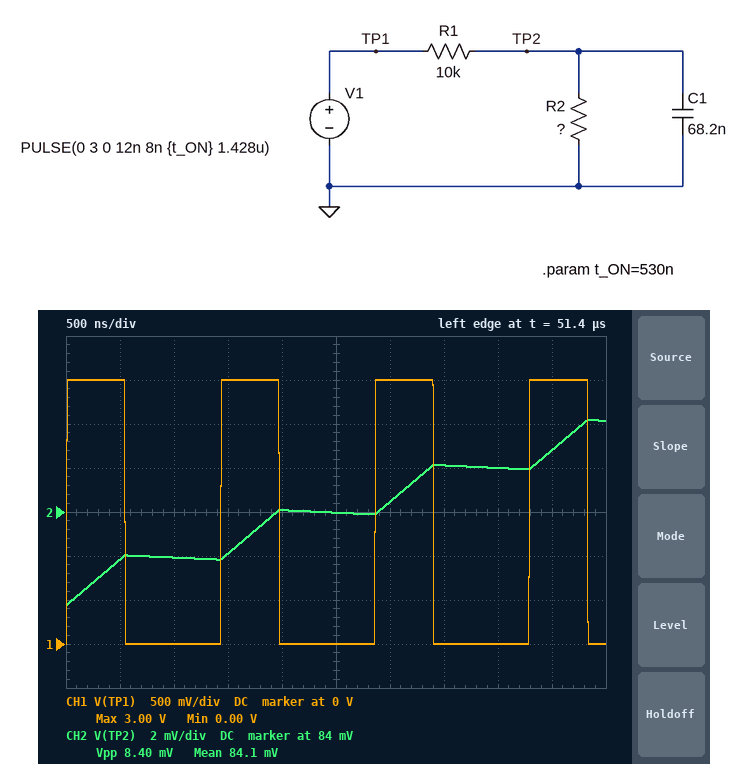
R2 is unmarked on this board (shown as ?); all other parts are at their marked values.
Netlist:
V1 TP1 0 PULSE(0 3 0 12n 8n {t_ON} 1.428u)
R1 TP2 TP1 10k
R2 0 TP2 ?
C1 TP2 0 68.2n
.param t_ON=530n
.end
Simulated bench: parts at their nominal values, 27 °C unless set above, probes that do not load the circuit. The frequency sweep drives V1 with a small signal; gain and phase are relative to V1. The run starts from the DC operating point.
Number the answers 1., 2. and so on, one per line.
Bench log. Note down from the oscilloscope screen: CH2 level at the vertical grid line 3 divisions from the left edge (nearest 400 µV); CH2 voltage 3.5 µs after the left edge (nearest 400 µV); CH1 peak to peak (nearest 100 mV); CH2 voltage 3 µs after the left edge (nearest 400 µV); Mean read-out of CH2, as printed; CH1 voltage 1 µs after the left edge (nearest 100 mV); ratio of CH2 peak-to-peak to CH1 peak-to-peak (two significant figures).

1. 82.0 mV
2. 86.0 mV
3. 3.0 V
4. 84.4 mV
5. 84.1 mV
6. 0 V
7. 0.0028
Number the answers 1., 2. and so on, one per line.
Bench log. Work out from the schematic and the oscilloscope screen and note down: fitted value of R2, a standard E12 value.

1. 12 kΩ
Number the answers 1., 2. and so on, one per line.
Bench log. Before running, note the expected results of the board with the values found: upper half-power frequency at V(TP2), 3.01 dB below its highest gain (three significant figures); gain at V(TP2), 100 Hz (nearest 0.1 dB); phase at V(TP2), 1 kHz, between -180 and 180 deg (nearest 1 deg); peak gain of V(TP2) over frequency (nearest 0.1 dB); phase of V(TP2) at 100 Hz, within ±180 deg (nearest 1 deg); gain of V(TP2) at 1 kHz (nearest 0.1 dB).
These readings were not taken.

1. 428 Hz
2. -5.5 dB
3. -67 deg
4. -5.3 dB
5. -13 deg
6. -13.4 dB
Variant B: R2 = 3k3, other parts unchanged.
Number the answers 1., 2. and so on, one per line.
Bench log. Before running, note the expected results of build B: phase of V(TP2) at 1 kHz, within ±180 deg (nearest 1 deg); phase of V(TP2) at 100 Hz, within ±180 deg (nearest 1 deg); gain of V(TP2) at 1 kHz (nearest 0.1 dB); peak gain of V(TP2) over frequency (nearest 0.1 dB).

1. -47 deg
2. -6 deg
3. -15.4 dB
4. -12.1 dB
